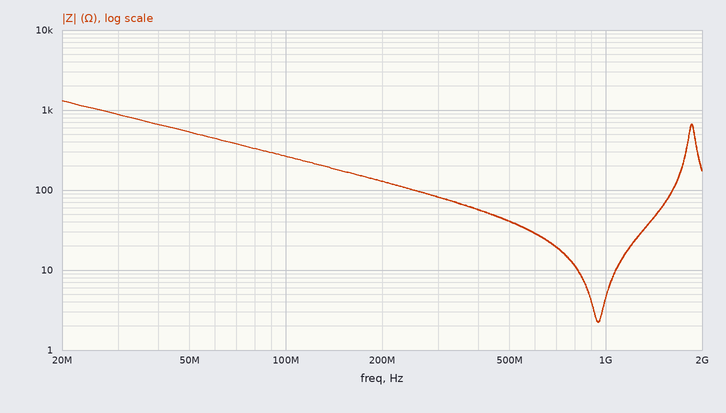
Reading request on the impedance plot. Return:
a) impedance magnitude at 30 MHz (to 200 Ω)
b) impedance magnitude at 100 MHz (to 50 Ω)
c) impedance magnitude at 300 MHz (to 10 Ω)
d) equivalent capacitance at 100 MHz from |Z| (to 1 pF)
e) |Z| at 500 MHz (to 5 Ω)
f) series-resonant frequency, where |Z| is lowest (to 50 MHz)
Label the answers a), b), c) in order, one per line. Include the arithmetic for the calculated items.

a) 800 Ω
b) 250 Ω
c) 80 Ω
d) C = 1/(2π × 100 MHz × 250 Ω) ≈ 6 pF
e) 40 Ω
f) 950 MHz
